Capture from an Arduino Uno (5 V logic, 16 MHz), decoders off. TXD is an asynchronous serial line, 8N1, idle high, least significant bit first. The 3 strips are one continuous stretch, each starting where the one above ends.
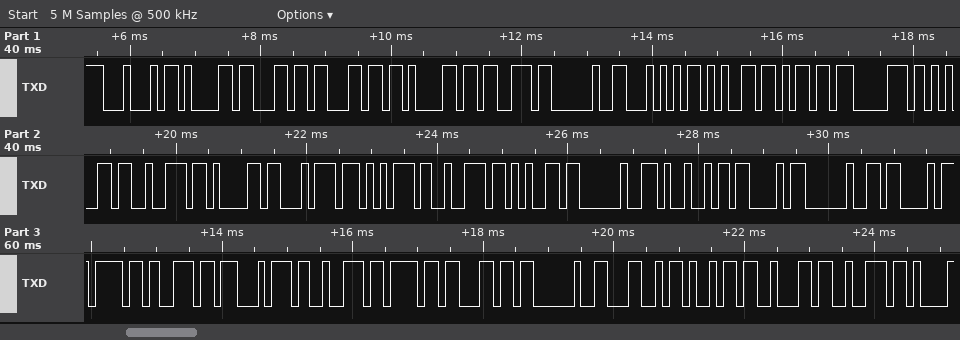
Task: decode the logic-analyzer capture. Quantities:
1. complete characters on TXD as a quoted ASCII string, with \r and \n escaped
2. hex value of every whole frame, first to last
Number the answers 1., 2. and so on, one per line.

1. "Dallas Temperature IC Control Libr"
2. 44 61 6C 6C 61 73 20 54 65 6D 70 65 72 61 74 75 72 65 20 49 43 20 43 6F 6E 74 72 6F 6C 20 4C 69 62 72
